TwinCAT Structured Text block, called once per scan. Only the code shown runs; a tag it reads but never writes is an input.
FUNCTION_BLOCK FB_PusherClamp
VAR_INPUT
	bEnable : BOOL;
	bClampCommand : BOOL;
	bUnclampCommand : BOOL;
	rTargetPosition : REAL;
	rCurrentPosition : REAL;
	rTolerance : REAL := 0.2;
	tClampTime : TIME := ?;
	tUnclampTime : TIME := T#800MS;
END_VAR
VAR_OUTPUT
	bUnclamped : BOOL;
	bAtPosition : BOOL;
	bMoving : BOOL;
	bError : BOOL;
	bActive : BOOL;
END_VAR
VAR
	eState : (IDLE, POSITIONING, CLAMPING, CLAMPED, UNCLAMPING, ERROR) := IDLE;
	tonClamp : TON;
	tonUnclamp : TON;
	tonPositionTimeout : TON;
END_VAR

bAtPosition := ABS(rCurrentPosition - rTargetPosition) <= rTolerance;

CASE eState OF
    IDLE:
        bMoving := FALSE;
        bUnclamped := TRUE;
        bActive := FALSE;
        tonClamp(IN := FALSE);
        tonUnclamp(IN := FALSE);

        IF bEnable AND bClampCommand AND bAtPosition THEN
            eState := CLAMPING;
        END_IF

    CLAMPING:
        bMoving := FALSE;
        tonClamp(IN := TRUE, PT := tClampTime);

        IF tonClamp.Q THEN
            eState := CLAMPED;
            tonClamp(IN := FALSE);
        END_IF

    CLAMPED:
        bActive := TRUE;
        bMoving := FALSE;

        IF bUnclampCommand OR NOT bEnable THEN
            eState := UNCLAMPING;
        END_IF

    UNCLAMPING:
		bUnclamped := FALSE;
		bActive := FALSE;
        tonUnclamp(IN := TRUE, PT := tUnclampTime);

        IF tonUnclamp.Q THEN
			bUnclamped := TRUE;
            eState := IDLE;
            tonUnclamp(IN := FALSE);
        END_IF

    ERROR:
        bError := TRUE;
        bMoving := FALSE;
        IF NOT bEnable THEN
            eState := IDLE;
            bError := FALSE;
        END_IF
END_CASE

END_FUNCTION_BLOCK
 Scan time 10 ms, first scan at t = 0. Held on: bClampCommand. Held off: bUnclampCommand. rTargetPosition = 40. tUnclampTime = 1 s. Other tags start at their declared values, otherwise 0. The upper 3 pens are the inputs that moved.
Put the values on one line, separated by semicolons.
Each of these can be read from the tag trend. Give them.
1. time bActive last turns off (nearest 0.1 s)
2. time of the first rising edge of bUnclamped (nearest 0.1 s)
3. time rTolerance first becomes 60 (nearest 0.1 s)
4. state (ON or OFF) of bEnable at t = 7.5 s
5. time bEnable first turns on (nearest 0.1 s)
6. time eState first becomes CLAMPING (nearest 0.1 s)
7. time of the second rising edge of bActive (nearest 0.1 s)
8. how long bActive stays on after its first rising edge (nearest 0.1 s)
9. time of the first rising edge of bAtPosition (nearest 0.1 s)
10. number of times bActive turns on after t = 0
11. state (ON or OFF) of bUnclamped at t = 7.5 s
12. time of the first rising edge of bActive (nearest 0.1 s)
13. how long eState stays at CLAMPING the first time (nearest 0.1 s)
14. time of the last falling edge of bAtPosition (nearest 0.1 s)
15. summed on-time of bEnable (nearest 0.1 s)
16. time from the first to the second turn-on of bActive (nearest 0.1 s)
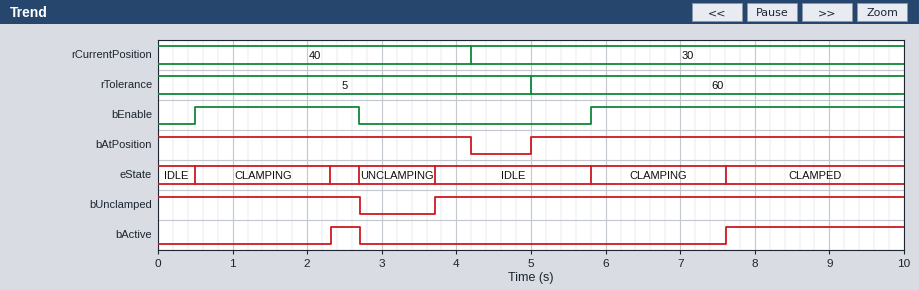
2.7 s; 3.7 s; 5.0 s; ON; 0.5 s; 0.5 s; 7.6 s; 0.4 s; 5.0 s; 2; ON; 2.3 s; 1.8 s; 4.2 s; 6.4 s; 5.3 s
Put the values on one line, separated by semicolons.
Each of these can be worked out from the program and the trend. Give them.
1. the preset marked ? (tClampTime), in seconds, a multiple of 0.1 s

1.8 s
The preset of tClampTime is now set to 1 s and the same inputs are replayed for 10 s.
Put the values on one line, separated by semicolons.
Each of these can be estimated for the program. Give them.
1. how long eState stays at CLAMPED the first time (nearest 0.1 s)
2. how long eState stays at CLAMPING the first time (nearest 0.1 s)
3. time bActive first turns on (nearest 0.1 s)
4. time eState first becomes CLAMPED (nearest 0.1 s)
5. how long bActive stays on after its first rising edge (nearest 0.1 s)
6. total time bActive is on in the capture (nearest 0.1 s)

1.2 s; 1.0 s; 1.5 s; 1.5 s; 1.2 s; 4.4 s
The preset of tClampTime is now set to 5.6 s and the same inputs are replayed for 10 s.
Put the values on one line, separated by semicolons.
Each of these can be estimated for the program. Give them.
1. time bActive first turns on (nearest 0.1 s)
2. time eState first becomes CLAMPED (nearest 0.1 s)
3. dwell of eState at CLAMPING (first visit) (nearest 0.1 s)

6.1 s; 6.1 s; 5.6 s
